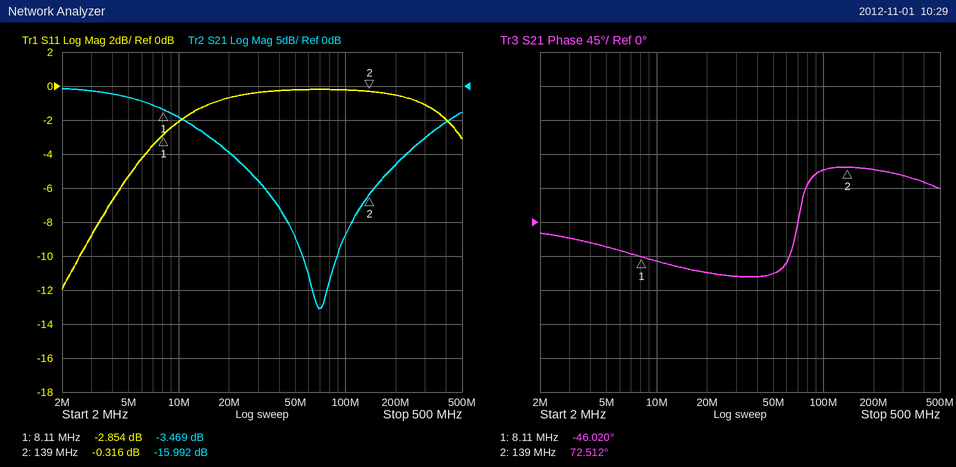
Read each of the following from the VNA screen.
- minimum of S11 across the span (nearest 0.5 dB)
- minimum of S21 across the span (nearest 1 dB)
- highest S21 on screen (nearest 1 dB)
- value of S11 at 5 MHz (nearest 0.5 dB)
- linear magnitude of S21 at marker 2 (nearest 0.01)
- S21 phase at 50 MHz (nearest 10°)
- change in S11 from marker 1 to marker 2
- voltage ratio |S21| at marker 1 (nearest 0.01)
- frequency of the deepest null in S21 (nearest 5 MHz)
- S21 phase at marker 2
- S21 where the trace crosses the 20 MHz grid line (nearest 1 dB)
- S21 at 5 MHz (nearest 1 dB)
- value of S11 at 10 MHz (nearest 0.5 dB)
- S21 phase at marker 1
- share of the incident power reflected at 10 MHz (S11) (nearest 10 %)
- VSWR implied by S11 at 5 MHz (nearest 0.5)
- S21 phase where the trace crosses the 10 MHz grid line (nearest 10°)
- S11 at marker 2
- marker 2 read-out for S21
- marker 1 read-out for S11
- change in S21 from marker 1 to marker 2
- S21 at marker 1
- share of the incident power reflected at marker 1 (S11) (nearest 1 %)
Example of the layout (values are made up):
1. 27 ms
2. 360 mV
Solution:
1. -12.0 dB
2. -33 dB
3. 0 dB
4. -5.5 dB
5. 0.16
6. -70°
7. 2.538 dB
8. 0.67
9. 70 MHz
10. 72.512°
11. -10 dB
12. -2 dB
13. -2.0 dB
14. -46.020°
15. 60 %
16. 3.5
17. -50°
18. -0.316 dB
19. -15.992 dB
20. -2.854 dB
21. -12.523 dB
22. -3.469 dB
23. 52 %
